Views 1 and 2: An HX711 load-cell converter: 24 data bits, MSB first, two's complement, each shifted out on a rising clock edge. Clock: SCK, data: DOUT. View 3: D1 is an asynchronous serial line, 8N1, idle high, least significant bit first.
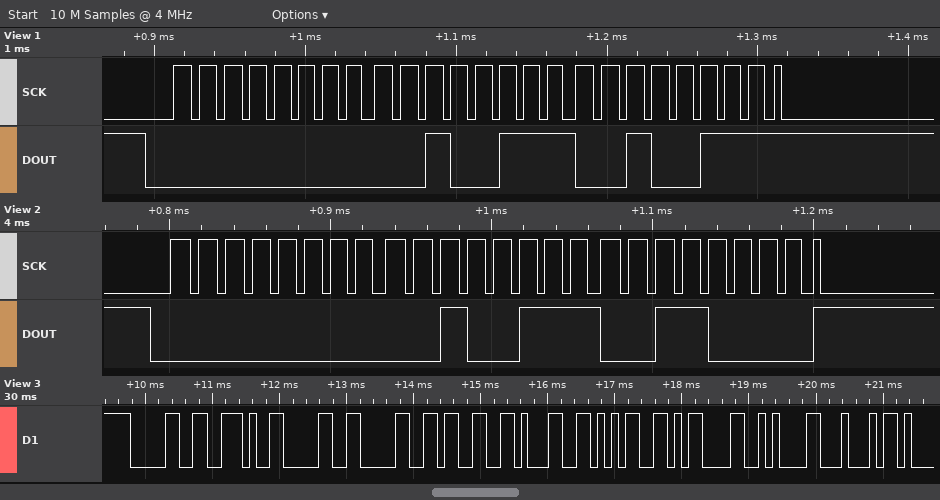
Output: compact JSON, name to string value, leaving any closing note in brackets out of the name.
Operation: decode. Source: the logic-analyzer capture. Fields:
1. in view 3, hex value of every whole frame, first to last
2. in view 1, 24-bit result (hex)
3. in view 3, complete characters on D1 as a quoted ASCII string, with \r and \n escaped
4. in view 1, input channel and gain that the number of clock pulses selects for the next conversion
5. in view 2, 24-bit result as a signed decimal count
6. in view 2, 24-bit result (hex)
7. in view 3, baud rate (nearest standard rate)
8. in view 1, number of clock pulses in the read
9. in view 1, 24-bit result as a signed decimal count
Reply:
{"in view 3, hex value of every whole frame, first to last": "0x30 0x2E 0x30 0x30 0x33 0x31 0x35 0x0D 0x0A 0x44", "in view 1, 24-bit result": "0x002727", "in view 3, complete characters on D1 as a quoted ASCII string, with \\r and \\n escaped": "\"0.00315\\r\\nD\"", "in view 1, input channel and gain that the number of clock pulses selects for the next conversion": "channel A, gain 128", "in view 2, 24-bit result as a signed decimal count": "10032", "in view 2, 24-bit result": "0x002730", "in view 3, baud rate": "9600 baud", "in view 1, number of clock pulses in the read": "25", "in view 1, 24-bit result as a signed decimal count": "10023"}
